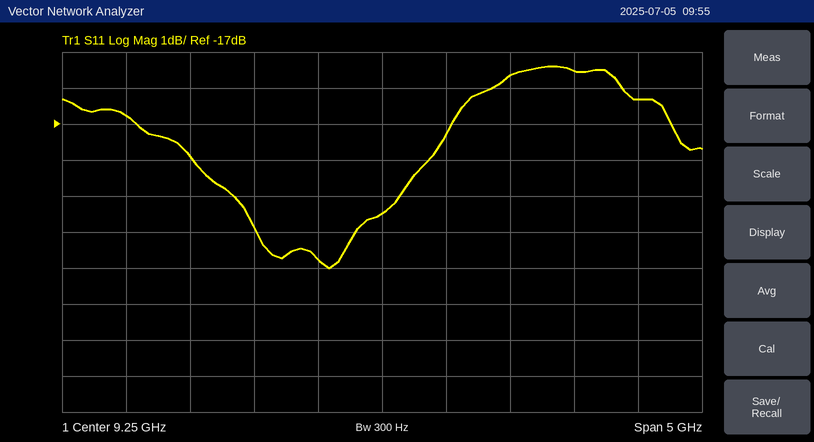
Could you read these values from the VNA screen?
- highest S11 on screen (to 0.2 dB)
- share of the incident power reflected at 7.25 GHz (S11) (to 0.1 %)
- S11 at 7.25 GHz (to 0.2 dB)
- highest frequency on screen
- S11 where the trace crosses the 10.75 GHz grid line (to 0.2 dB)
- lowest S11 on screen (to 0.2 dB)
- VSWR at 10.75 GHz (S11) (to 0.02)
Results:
-15.4 dB
2.1 %
-16.8 dB
11.75 GHz
-15.6 dB
-21.0 dB
1.40
